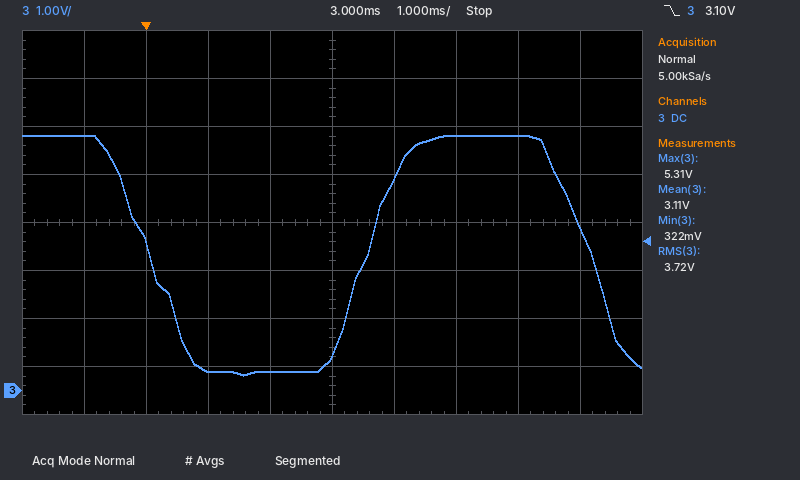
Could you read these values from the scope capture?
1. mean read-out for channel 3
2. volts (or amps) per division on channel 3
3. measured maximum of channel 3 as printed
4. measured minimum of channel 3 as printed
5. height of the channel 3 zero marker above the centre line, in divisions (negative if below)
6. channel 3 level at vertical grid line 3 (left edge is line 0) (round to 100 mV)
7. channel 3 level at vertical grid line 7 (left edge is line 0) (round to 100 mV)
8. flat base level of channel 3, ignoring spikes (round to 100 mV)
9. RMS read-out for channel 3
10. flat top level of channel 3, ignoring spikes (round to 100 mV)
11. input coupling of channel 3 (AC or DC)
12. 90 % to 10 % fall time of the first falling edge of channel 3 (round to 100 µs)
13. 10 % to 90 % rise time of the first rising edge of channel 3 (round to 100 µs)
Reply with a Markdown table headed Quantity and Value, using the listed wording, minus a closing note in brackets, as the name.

| Quantity | Value |
|---|---|
| mean read-out for channel 3 | 3.11 V |
| volts (or amps) per division on channel 3 | 1 V |
| measured maximum of channel 3 as printed | 5.31 V |
| measured minimum of channel 3 as printed | 322 mV |
| height of the channel 3 zero marker above the centre line, in divisions | -3.5 div |
| channel 3 level at vertical grid line 3 (left edge is line 0) | 400 mV |
| channel 3 level at vertical grid line 7 (left edge is line 0) | 5.3 V |
| flat base level of channel 3, ignoring spikes | 400 mV |
| RMS read-out for channel 3 | 3.72 V |
| flat top level of channel 3, ignoring spikes | 5.3 V |
| input coupling of channel 3 | DC |
| 90 % to 10 % fall time of the first falling edge of channel 3 | 1.2 ms |
| 10 % to 90 % rise time of the first rising edge of channel 3 | 1.1 ms |
